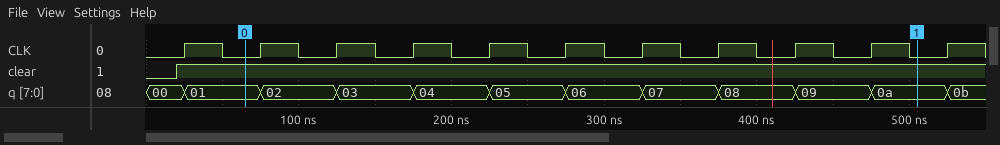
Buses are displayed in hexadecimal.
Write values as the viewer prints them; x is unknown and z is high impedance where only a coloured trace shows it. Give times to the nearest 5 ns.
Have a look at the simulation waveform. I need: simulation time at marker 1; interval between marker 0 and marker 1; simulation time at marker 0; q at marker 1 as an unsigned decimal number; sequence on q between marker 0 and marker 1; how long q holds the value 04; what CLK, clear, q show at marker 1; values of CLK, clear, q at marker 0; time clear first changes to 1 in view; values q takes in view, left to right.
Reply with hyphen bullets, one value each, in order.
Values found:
- 505 ns
- 440 ns
- 65 ns
- 10
- 01, 02, 03, 04, 05, 06, 07, 08, 09, 0a
- 50 ns
- CLK=0, clear=1, q=0a
- CLK=0, clear=1, q=01
- 20 ns
- 00, 01, 02, 03, 04, 05, 06, 07, 08, 09, 0a, 0b
